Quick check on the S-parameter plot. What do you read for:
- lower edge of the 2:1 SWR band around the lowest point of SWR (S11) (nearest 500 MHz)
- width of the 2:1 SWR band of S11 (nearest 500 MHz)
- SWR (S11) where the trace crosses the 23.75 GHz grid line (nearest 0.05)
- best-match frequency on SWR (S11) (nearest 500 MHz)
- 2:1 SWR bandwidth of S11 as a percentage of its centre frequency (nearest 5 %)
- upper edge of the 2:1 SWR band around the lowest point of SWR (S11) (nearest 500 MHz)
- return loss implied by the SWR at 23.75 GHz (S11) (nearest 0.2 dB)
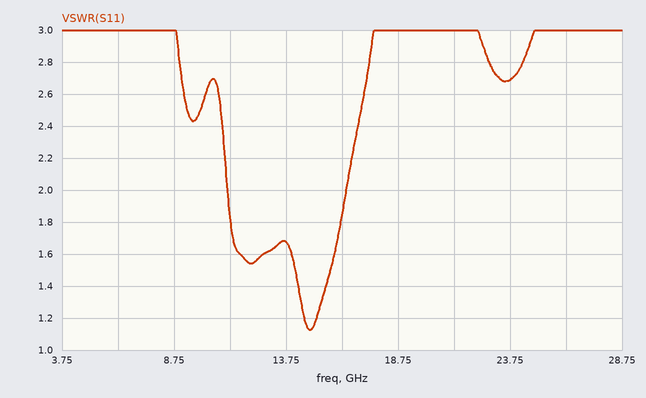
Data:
11.0 GHz
5.5 GHz
2.70
15.0 GHz
40 %
16.5 GHz
6.8 dB
